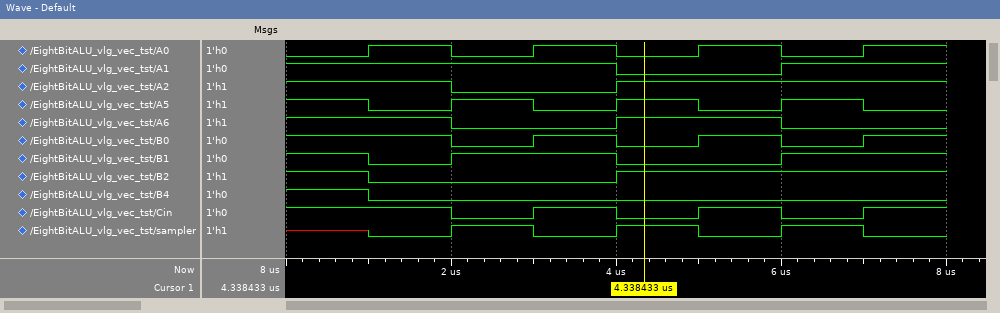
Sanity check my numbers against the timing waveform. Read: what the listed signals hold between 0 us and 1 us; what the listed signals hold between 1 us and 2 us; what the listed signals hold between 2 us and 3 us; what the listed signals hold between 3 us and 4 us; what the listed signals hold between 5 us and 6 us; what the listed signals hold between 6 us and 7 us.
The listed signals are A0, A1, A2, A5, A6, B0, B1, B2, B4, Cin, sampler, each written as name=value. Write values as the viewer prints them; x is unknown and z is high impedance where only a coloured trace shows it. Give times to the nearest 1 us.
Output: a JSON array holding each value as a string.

["A0=0, A1=1, A2=1, A5=1, A6=1, B0=1, B1=1, B2=1, B4=1, Cin=1, sampler=x", "A0=1, A1=1, A2=1, A5=0, A6=1, B0=1, B1=0, B2=0, B4=0, Cin=1, sampler=0", "A0=0, A1=1, A2=0, A5=1, A6=0, B0=0, B1=1, B2=0, B4=0, Cin=0, sampler=1", "A0=1, A1=1, A2=0, A5=0, A6=0, B0=1, B1=1, B2=0, B4=0, Cin=1, sampler=0", "A0=1, A1=0, A2=1, A5=0, A6=1, B0=1, B1=0, B2=1, B4=0, Cin=1, sampler=0", "A0=0, A1=1, A2=1, A5=1, A6=0, B0=0, B1=1, B2=1, B4=0, Cin=0, sampler=1"]
